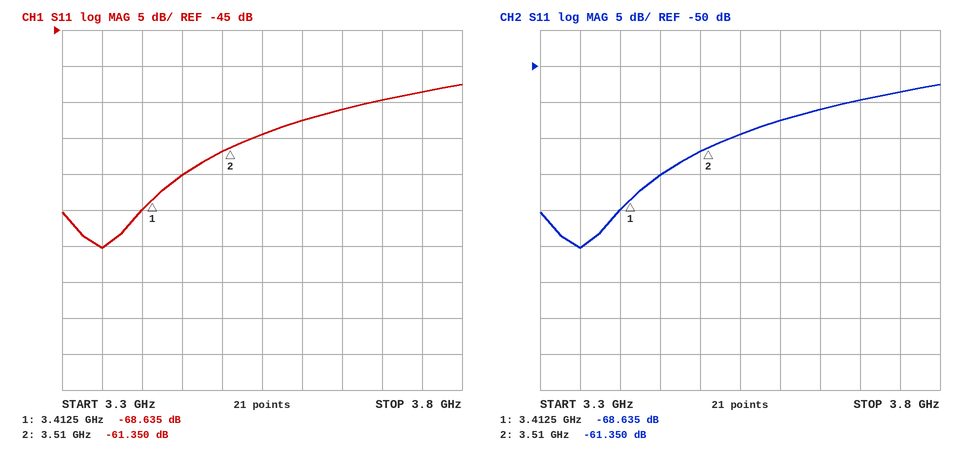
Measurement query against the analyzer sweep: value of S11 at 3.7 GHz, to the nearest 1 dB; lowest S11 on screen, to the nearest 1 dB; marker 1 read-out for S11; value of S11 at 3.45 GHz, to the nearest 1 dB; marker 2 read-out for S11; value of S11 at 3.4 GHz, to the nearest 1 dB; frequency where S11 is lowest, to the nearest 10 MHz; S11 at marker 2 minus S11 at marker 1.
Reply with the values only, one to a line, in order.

-55 dB
-75 dB
-68.635 dB
-65 dB
-61.350 dB
-70 dB
3.35 GHz
7.285 dB
